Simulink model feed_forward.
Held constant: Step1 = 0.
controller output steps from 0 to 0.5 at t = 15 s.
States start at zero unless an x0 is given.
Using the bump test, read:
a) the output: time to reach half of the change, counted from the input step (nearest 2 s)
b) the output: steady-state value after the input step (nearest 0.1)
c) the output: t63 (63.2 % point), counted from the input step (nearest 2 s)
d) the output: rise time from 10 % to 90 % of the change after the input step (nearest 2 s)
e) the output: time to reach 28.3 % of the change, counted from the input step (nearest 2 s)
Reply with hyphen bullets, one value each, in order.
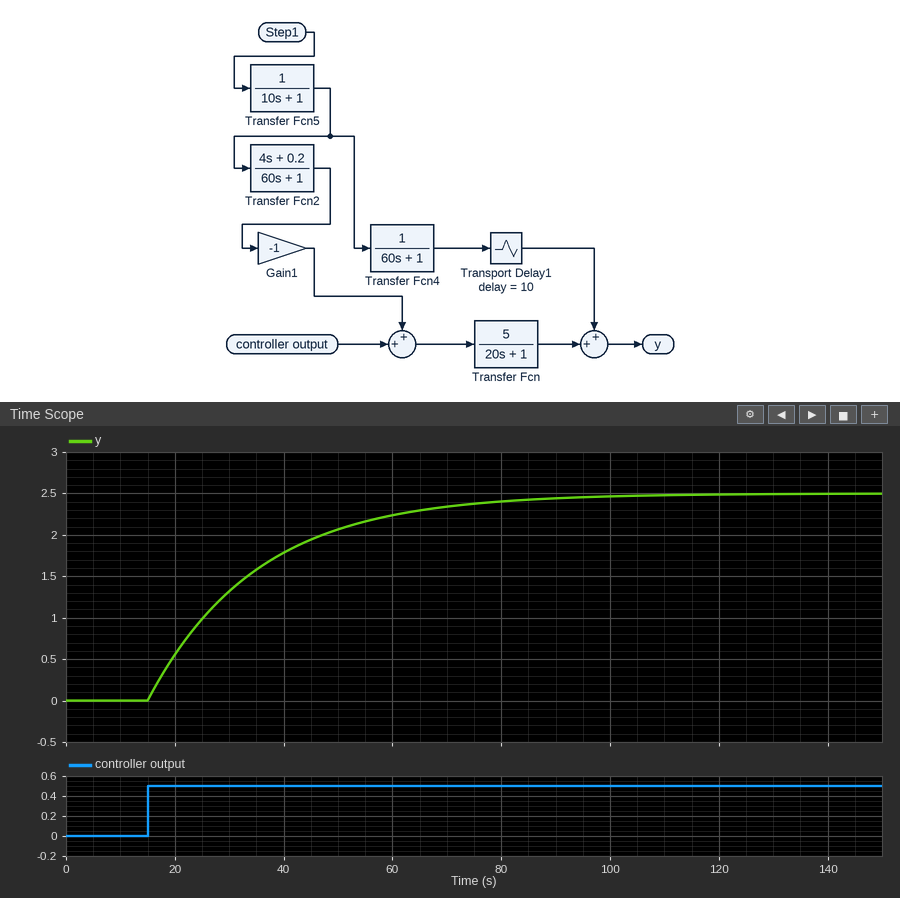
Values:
- 14 s
- 2.5
- 20 s
- 44 s
- 6 s
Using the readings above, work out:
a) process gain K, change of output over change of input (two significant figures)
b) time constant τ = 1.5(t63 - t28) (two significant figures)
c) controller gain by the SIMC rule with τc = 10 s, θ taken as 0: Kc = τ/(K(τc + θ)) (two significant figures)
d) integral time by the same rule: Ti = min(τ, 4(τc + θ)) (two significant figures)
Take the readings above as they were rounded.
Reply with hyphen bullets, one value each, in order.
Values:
- 5.0
- 21 s
- 0.42
- 21 s
